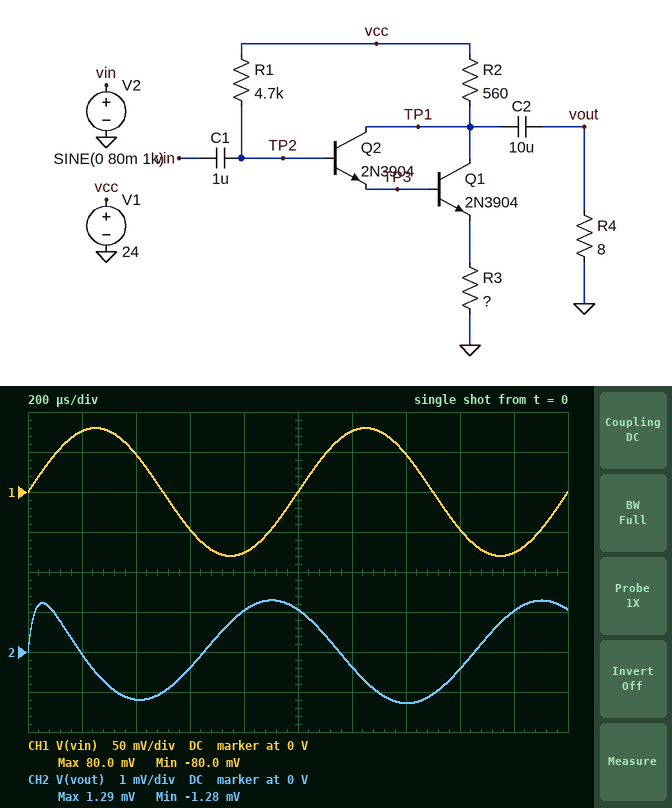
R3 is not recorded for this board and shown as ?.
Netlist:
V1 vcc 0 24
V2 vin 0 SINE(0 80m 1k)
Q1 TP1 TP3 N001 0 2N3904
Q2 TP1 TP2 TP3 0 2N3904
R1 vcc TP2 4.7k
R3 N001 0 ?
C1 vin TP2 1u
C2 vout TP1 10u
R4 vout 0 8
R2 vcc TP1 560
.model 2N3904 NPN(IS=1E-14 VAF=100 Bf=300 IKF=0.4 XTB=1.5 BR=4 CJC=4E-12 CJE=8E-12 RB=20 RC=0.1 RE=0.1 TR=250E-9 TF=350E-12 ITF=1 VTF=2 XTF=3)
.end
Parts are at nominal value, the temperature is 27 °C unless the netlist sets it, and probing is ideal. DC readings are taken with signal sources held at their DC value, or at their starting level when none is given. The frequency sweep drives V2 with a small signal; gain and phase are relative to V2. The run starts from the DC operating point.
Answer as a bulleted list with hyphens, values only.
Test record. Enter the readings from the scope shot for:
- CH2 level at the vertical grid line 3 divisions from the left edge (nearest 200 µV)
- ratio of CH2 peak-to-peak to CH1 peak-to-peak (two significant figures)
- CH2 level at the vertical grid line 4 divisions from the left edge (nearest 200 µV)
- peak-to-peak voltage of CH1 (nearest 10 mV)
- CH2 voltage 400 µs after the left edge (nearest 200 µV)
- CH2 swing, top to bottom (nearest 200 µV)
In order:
- -400 µV
- 0.016
- 1.0 mV
- 160 mV
- -1.2 mV
- 2.6 mV
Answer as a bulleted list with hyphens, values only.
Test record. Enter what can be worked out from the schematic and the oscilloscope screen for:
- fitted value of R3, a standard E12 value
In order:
- 6.8 Ω
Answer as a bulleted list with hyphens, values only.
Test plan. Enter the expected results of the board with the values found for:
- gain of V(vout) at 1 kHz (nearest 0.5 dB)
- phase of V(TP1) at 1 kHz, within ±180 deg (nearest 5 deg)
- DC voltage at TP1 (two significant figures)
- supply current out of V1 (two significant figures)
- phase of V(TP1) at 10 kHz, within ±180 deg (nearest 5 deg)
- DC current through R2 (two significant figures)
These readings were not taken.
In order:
- -36.0 dB
- 60 deg
- 1.1 V
- 46 mA
- 25 deg
- 41 mA
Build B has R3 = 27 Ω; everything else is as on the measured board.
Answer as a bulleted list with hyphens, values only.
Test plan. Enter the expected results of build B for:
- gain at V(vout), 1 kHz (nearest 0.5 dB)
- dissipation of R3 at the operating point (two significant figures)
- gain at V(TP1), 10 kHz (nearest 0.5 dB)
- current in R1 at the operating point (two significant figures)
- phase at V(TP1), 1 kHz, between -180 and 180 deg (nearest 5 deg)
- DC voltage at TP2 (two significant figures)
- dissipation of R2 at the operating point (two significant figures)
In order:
- -30.0 dB
- 52 mW
- -15.5 dB
- 4.5 mA
- 40 deg
- 2.8 V
- 870 mW
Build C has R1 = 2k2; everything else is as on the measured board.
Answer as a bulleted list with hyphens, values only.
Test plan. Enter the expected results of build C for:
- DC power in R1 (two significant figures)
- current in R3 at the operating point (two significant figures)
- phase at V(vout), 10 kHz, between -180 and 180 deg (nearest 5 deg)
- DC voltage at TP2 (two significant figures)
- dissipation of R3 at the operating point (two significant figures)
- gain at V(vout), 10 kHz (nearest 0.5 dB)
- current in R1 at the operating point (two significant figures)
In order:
- 220 mW
- 51 mA
- 40 deg
- 2.1 V
- 18 mW
- -18.5 dB
- 10 mA
